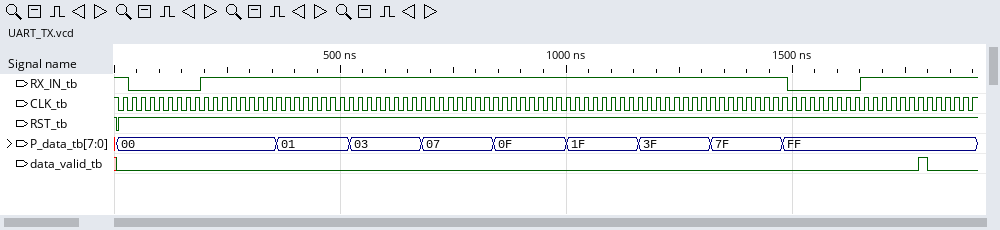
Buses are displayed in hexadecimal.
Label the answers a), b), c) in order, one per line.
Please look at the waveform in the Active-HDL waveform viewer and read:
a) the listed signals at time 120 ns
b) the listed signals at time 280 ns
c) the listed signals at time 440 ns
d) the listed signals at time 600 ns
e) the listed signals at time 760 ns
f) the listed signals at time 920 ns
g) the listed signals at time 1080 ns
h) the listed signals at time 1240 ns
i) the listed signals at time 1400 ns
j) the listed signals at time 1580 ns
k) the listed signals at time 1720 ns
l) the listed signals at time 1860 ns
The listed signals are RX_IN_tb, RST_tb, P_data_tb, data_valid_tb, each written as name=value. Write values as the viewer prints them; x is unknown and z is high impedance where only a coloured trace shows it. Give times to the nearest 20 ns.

a) RX_IN_tb=0, RST_tb=1, P_data_tb=00, data_valid_tb=0
b) RX_IN_tb=1, RST_tb=1, P_data_tb=00, data_valid_tb=0
c) RX_IN_tb=1, RST_tb=1, P_data_tb=01, data_valid_tb=0
d) RX_IN_tb=1, RST_tb=1, P_data_tb=03, data_valid_tb=0
e) RX_IN_tb=1, RST_tb=1, P_data_tb=07, data_valid_tb=0
f) RX_IN_tb=1, RST_tb=1, P_data_tb=0F, data_valid_tb=0
g) RX_IN_tb=1, RST_tb=1, P_data_tb=1F, data_valid_tb=0
h) RX_IN_tb=1, RST_tb=1, P_data_tb=3F, data_valid_tb=0
i) RX_IN_tb=1, RST_tb=1, P_data_tb=7F, data_valid_tb=0
j) RX_IN_tb=0, RST_tb=1, P_data_tb=FF, data_valid_tb=0
k) RX_IN_tb=1, RST_tb=1, P_data_tb=FF, data_valid_tb=0
l) RX_IN_tb=1, RST_tb=1, P_data_tb=FF, data_valid_tb=0
